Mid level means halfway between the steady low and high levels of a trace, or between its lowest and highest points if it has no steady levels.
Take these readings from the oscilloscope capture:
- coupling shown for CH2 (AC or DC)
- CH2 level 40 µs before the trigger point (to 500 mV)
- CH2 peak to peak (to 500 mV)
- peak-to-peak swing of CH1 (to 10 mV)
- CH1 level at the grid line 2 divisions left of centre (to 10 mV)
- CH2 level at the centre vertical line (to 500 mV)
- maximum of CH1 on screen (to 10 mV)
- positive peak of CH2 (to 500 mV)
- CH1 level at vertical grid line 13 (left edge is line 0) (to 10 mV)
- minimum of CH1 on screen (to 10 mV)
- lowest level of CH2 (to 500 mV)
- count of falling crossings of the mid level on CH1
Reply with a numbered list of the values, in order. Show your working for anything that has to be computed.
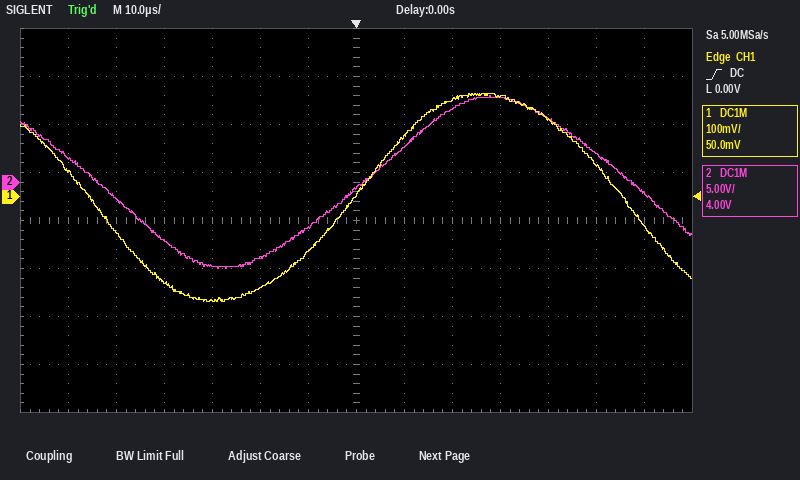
1. DC
2. -6.0 V
3. 9.0 V − (-9.0 V) = 18.0 V
4. 210 mV − (-220 mV) = 430 mV
5. -190 mV
6. -500 mV
7. 210 mV
8. 9.0 V
9. -60 mV
10. -220 mV
11. -9.0 V
12. 2
